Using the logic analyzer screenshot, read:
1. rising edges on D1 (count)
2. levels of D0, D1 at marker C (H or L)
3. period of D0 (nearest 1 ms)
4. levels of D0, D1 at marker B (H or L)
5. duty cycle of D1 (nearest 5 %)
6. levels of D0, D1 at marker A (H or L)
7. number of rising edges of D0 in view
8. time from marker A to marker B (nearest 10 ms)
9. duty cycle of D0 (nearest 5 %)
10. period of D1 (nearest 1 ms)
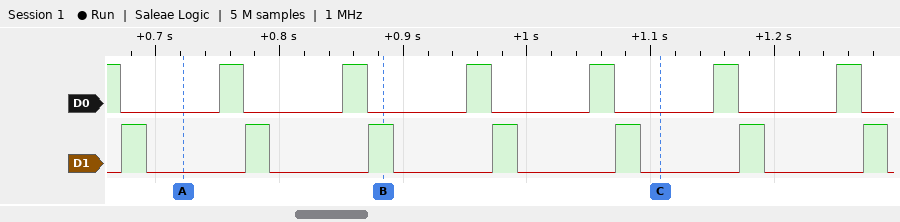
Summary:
7
D0=L, D1=L
100 ms
D0=L, D1=H
20 %
D0=L, D1=L
6
160 ms
20 %
100 ms
